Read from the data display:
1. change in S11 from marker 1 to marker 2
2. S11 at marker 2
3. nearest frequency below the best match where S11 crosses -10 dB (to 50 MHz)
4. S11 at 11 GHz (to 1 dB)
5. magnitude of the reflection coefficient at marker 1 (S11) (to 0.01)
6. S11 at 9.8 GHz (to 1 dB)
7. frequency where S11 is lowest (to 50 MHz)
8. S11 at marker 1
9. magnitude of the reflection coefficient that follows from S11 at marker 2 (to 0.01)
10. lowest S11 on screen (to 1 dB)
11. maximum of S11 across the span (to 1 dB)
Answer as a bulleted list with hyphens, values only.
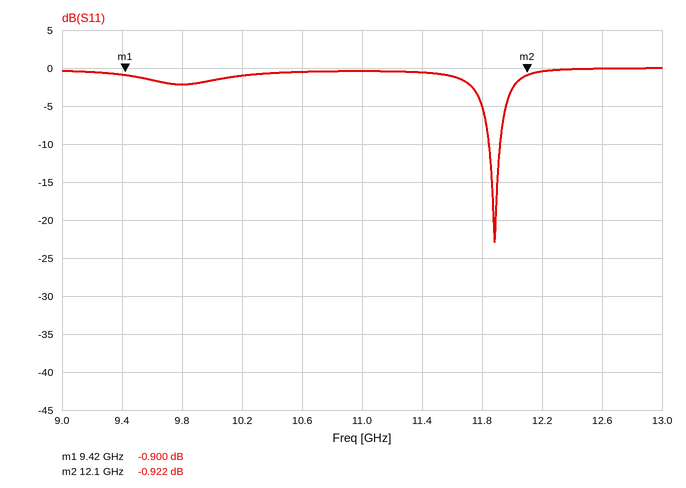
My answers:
- -0.022 dB
- -0.922 dB
- 11.85 GHz
- 0 dB
- 0.90
- -2 dB
- 11.90 GHz
- -0.900 dB
- 0.90
- -23 dB
- 0 dB
